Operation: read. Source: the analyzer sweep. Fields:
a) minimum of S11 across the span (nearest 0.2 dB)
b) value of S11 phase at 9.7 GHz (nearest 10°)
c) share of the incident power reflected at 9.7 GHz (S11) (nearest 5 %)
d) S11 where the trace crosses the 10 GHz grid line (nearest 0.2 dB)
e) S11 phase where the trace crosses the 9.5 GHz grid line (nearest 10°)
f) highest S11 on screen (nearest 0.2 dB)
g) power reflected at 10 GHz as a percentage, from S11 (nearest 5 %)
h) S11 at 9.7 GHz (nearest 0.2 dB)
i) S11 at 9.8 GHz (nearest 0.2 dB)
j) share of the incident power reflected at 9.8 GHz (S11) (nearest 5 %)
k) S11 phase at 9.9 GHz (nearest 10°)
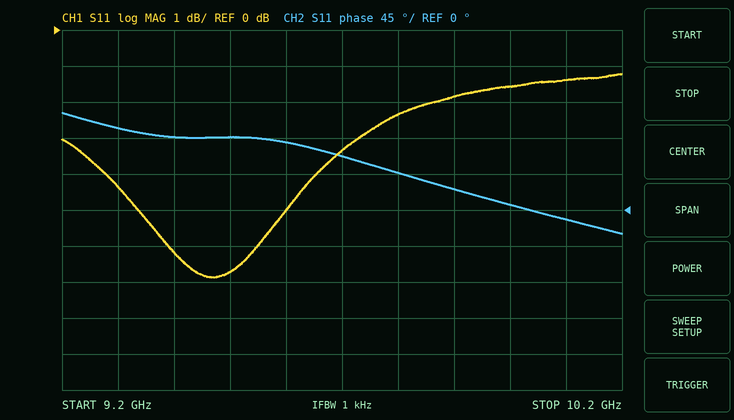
-6.8 dB
70°
45 %
-1.6 dB
90°
-1.2 dB
70 %
-3.4 dB
-2.4 dB
60 %
30°
